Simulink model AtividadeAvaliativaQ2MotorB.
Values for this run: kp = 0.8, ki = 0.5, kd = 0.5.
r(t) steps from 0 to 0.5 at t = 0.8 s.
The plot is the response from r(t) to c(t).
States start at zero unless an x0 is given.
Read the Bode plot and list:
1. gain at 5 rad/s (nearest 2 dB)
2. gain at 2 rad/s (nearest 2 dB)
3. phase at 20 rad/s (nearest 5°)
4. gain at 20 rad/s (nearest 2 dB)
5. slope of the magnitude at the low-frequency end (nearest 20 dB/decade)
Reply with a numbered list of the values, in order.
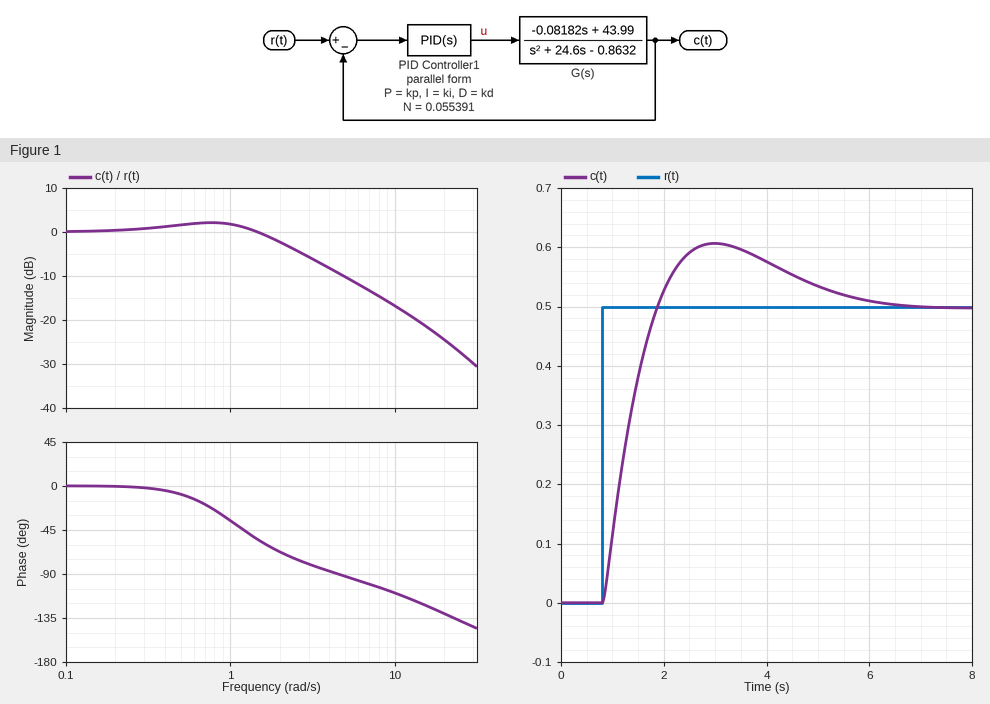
1. -10 dB
2. -2 dB
3. -130°
4. -24 dB
5. 0 dB/decade
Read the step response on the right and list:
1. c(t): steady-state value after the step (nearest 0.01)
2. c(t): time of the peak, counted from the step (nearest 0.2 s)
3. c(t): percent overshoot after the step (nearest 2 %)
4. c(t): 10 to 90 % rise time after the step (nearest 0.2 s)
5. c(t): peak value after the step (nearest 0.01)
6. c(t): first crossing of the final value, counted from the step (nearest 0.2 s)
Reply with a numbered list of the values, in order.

1. 0.50
2. 2.2 s
3. 22 %
4. 0.8 s
5. 0.61
6. 1.0 s
